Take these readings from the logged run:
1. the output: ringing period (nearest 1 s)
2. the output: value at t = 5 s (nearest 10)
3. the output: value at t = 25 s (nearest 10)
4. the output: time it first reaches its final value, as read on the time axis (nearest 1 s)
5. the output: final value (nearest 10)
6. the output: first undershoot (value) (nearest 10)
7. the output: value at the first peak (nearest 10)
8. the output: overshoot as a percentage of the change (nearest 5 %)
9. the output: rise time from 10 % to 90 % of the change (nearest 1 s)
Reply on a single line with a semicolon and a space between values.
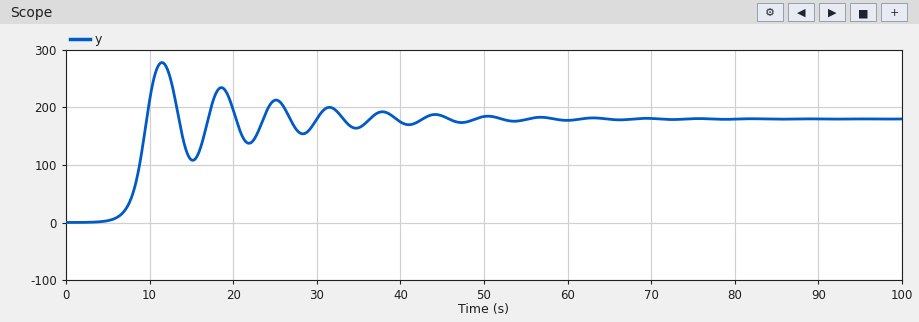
7 s; 0; 210; 10 s; 180; 110; 280; 55 %; 3 s
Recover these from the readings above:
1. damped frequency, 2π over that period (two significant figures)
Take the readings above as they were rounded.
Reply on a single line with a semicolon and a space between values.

0.90 rad/s
